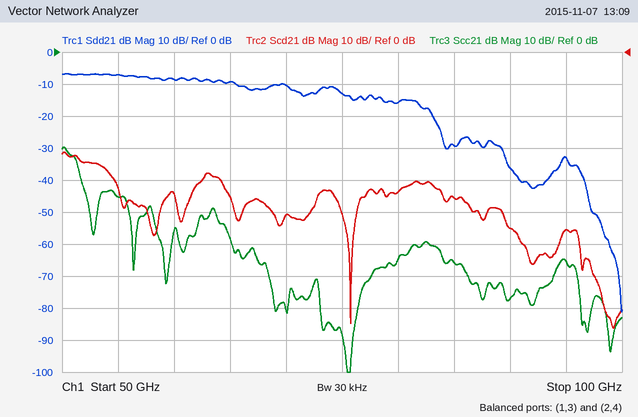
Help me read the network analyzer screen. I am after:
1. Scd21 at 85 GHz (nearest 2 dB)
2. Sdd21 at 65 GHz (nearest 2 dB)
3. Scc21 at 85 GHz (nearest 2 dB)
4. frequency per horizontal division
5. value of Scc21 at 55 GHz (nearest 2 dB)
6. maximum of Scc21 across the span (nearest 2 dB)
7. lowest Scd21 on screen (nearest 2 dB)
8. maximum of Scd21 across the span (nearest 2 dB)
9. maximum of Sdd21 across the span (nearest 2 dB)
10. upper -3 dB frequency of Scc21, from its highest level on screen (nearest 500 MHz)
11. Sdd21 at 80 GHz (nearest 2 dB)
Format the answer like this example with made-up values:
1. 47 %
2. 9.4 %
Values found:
1. -46 dB
2. -10 dB
3. -66 dB
4. 5 GHz
5. -46 dB
6. -30 dB
7. -86 dB
8. -32 dB
9. -6 dB
10. 51.0 GHz
11. -16 dB
